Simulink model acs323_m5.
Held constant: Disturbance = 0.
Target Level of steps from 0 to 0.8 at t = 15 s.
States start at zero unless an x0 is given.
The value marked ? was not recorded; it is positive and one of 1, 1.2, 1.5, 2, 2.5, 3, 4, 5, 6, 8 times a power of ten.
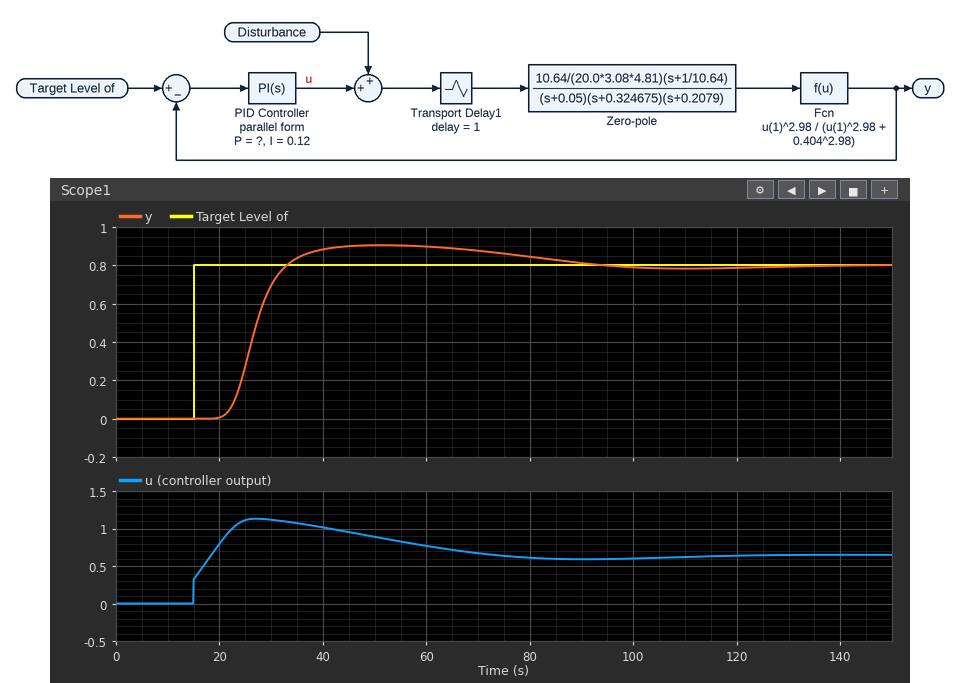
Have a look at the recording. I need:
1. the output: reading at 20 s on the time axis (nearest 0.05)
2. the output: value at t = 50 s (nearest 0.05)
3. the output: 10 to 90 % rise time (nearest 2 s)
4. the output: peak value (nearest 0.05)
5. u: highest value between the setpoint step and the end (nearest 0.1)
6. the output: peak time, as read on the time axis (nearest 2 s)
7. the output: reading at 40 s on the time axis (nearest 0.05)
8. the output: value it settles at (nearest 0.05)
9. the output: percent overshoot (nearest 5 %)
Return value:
0.00
0.90
8 s
0.90
1.1
52 s
0.90
0.80
15 %
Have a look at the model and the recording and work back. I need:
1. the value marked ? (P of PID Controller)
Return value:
0.4
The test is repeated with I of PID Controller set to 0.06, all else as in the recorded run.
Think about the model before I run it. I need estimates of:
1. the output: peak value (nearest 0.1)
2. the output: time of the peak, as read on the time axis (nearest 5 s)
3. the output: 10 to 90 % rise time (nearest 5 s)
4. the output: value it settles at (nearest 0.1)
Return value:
0.8
75 s
15 s
0.8
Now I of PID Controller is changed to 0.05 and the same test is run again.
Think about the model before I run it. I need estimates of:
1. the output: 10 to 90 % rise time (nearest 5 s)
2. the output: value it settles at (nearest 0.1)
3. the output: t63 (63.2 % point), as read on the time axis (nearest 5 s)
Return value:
20 s
0.8
35 s
